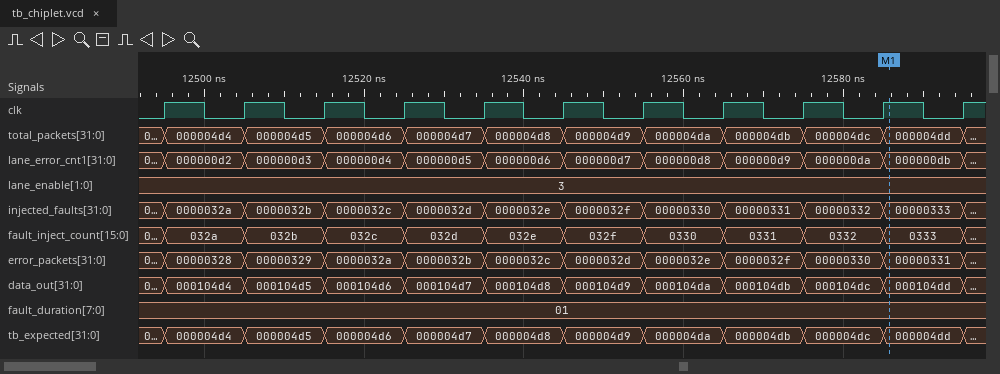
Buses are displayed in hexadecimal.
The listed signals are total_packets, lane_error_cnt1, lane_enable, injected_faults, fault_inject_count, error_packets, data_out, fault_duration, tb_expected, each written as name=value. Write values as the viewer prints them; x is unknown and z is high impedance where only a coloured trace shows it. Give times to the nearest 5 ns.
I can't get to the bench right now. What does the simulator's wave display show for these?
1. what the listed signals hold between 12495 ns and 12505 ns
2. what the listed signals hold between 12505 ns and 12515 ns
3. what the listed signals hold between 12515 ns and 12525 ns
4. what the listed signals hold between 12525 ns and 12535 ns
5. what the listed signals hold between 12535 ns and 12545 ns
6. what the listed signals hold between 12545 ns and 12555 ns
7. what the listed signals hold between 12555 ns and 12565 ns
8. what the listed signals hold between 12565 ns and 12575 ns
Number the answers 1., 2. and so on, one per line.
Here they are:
1. total_packets=000004d4, lane_error_cnt1=000000d2, lane_enable=3, injected_faults=0000032a, fault_inject_count=032a, error_packets=00000328, data_out=000104d4, fault_duration=01, tb_expected=000004d4
2. total_packets=000004d5, lane_error_cnt1=000000d3, lane_enable=3, injected_faults=0000032b, fault_inject_count=032b, error_packets=00000329, data_out=000104d5, fault_duration=01, tb_expected=000004d5
3. total_packets=000004d6, lane_error_cnt1=000000d4, lane_enable=3, injected_faults=0000032c, fault_inject_count=032c, error_packets=0000032a, data_out=000104d6, fault_duration=01, tb_expected=000004d6
4. total_packets=000004d7, lane_error_cnt1=000000d5, lane_enable=3, injected_faults=0000032d, fault_inject_count=032d, error_packets=0000032b, data_out=000104d7, fault_duration=01, tb_expected=000004d7
5. total_packets=000004d8, lane_error_cnt1=000000d6, lane_enable=3, injected_faults=0000032e, fault_inject_count=032e, error_packets=0000032c, data_out=000104d8, fault_duration=01, tb_expected=000004d8
6. total_packets=000004d9, lane_error_cnt1=000000d7, lane_enable=3, injected_faults=0000032f, fault_inject_count=032f, error_packets=0000032d, data_out=000104d9, fault_duration=01, tb_expected=000004d9
7. total_packets=000004da, lane_error_cnt1=000000d8, lane_enable=3, injected_faults=00000330, fault_inject_count=0330, error_packets=0000032e, data_out=000104da, fault_duration=01, tb_expected=000004da
8. total_packets=000004db, lane_error_cnt1=000000d9, lane_enable=3, injected_faults=00000331, fault_inject_count=0331, error_packets=0000032f, data_out=000104db, fault_duration=01, tb_expected=000004db
